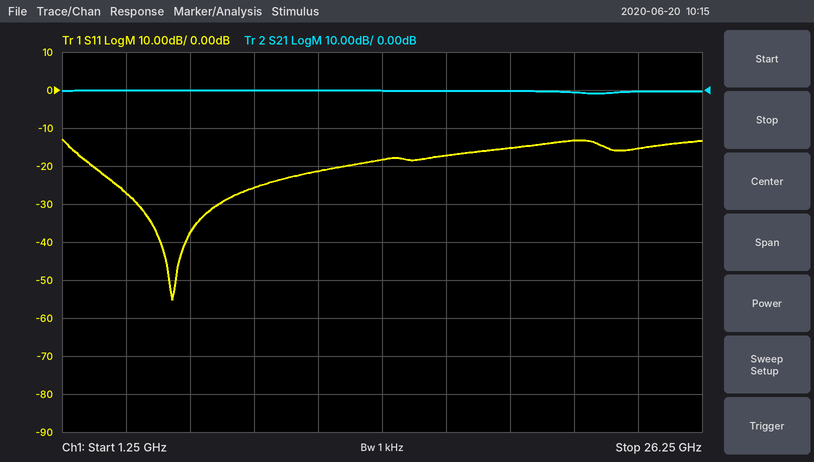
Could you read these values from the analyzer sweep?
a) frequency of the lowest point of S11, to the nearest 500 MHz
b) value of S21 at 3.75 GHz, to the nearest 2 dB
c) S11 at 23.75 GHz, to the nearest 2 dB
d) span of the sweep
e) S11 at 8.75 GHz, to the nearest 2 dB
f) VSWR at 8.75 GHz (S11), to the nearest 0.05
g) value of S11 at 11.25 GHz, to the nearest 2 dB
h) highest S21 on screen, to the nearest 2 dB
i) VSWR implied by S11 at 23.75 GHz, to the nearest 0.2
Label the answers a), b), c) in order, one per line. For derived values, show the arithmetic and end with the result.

a) 5.5 GHz
b) 0 dB
c) -16 dB
d) 25 GHz
e) -26 dB
f) |Γ| = 10^(-26/20) = 0.0501; VSWR = (1 + 0.0501)/(1 − 0.0501) ≈ 1.11, so 1.10 to the nearest 0.05
g) -22 dB
h) 0 dB
i) |Γ| = 10^(-16/20) = 0.1585; VSWR = (1 + 0.1585)/(1 − 0.1585) ≈ 1.4
